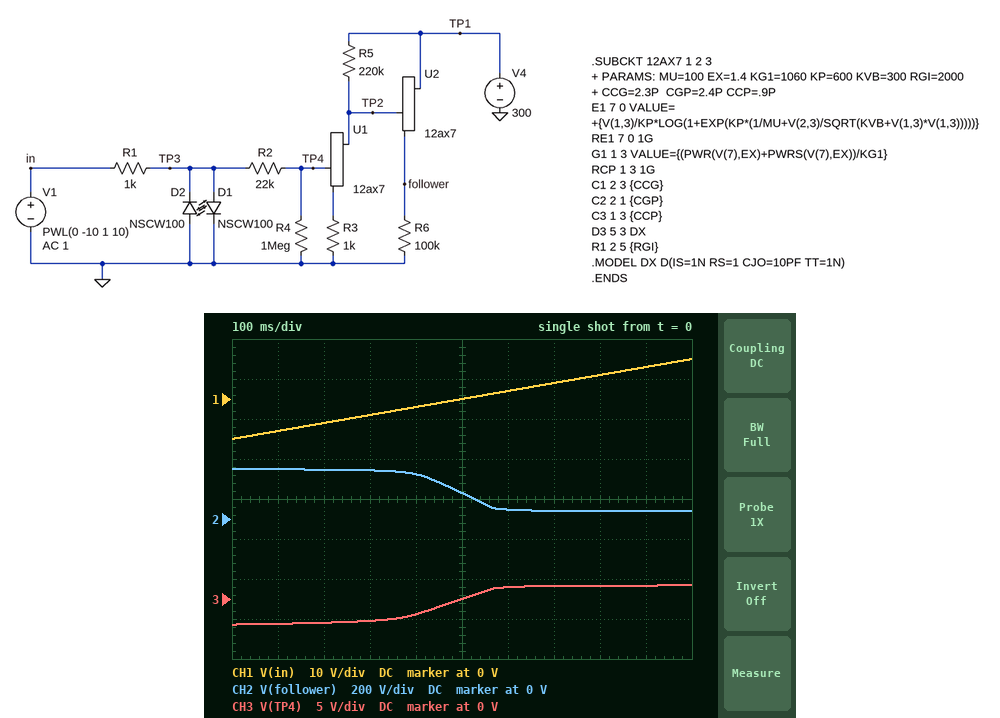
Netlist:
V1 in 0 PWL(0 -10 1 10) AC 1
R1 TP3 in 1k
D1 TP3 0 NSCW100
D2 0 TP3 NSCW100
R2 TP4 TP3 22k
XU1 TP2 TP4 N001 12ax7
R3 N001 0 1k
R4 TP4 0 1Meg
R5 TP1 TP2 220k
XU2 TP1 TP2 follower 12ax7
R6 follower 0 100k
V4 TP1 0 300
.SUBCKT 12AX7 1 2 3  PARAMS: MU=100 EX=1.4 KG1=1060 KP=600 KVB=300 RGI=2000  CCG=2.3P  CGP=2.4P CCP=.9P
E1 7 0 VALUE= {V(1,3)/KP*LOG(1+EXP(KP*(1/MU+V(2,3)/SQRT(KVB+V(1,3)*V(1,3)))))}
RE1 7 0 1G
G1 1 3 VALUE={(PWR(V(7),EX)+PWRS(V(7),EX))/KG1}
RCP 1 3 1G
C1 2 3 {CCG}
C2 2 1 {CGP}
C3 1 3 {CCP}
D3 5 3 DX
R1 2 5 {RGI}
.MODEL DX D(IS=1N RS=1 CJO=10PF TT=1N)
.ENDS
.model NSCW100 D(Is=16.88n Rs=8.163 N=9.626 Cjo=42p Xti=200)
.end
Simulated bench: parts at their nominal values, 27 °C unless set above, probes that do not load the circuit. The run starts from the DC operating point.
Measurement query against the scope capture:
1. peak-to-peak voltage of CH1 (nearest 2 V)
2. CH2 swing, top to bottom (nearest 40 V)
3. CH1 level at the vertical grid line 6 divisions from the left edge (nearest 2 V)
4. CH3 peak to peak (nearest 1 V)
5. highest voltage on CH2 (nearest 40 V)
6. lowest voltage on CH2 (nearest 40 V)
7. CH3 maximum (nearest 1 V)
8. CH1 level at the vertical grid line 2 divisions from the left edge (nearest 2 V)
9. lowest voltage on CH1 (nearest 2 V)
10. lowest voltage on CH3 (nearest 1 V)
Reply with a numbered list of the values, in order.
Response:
1. 20 V
2. 200 V
3. 2 V
4. 5 V
5. 240 V
6. 40 V
7. 2 V
8. -6 V
9. -10 V
10. -3 V
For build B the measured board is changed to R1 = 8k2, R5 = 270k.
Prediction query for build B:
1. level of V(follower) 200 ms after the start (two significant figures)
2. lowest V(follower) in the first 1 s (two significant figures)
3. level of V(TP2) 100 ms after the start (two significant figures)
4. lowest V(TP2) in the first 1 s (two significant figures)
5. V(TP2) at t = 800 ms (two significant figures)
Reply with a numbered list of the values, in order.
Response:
1. 230 V
2. 33 V
3. 240 V
4. 31 V
5. 32 V
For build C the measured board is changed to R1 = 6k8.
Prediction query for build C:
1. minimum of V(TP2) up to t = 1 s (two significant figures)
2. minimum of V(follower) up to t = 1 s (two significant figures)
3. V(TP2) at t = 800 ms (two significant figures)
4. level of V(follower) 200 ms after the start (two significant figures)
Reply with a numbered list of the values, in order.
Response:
1. 39 V
2. 41 V
3. 40 V
4. 240 V
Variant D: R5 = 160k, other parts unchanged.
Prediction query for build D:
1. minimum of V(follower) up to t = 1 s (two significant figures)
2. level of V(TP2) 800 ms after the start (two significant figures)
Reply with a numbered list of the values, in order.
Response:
1. 54 V
2. 53 V
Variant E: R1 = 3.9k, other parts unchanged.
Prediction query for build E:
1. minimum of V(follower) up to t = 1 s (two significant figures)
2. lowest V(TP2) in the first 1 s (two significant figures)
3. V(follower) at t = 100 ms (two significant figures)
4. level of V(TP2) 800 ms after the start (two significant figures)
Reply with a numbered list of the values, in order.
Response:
1. 40 V
2. 38 V
3. 240 V
4. 39 V
